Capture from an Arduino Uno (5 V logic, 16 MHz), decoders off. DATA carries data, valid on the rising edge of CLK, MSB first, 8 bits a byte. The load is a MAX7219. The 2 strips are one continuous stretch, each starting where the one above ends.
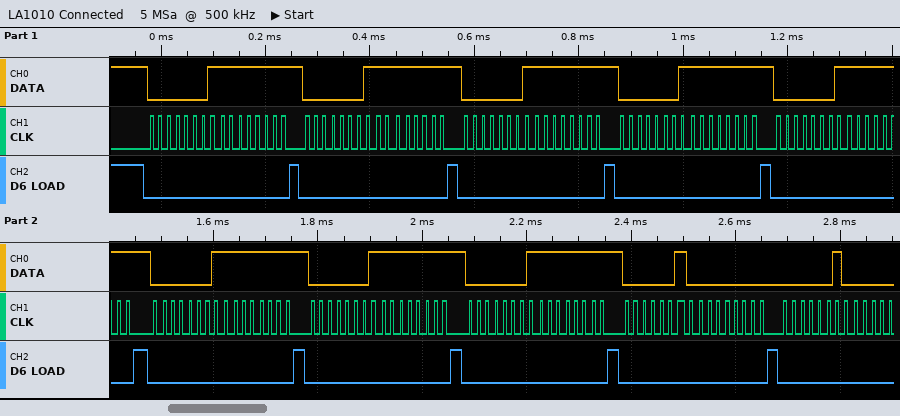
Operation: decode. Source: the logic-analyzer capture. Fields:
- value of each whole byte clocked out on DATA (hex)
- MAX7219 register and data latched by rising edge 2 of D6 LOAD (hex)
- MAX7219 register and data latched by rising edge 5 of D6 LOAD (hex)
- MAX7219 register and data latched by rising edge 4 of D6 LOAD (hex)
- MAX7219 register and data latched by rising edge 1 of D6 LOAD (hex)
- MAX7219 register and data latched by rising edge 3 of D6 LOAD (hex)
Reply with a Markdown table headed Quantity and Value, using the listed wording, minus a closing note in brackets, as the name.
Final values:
| Quantity | Value |
|---|---|
| value of each whole byte clocked out on DATA | 01 FF 01 FF 01 FF 01 FF 01 FF 01 FF 01 FF 01 FF 02 00 02 |
| MAX7219 register and data latched by rising edge 2 of D6 LOAD | register 0x1, data 0xFF |
| MAX7219 register and data latched by rising edge 5 of D6 LOAD | register 0x1, data 0xFF |
| MAX7219 register and data latched by rising edge 4 of D6 LOAD | register 0x1, data 0xFF |
| MAX7219 register and data latched by rising edge 1 of D6 LOAD | register 0x1, data 0xFF |
| MAX7219 register and data latched by rising edge 3 of D6 LOAD | register 0x1, data 0xFF |
